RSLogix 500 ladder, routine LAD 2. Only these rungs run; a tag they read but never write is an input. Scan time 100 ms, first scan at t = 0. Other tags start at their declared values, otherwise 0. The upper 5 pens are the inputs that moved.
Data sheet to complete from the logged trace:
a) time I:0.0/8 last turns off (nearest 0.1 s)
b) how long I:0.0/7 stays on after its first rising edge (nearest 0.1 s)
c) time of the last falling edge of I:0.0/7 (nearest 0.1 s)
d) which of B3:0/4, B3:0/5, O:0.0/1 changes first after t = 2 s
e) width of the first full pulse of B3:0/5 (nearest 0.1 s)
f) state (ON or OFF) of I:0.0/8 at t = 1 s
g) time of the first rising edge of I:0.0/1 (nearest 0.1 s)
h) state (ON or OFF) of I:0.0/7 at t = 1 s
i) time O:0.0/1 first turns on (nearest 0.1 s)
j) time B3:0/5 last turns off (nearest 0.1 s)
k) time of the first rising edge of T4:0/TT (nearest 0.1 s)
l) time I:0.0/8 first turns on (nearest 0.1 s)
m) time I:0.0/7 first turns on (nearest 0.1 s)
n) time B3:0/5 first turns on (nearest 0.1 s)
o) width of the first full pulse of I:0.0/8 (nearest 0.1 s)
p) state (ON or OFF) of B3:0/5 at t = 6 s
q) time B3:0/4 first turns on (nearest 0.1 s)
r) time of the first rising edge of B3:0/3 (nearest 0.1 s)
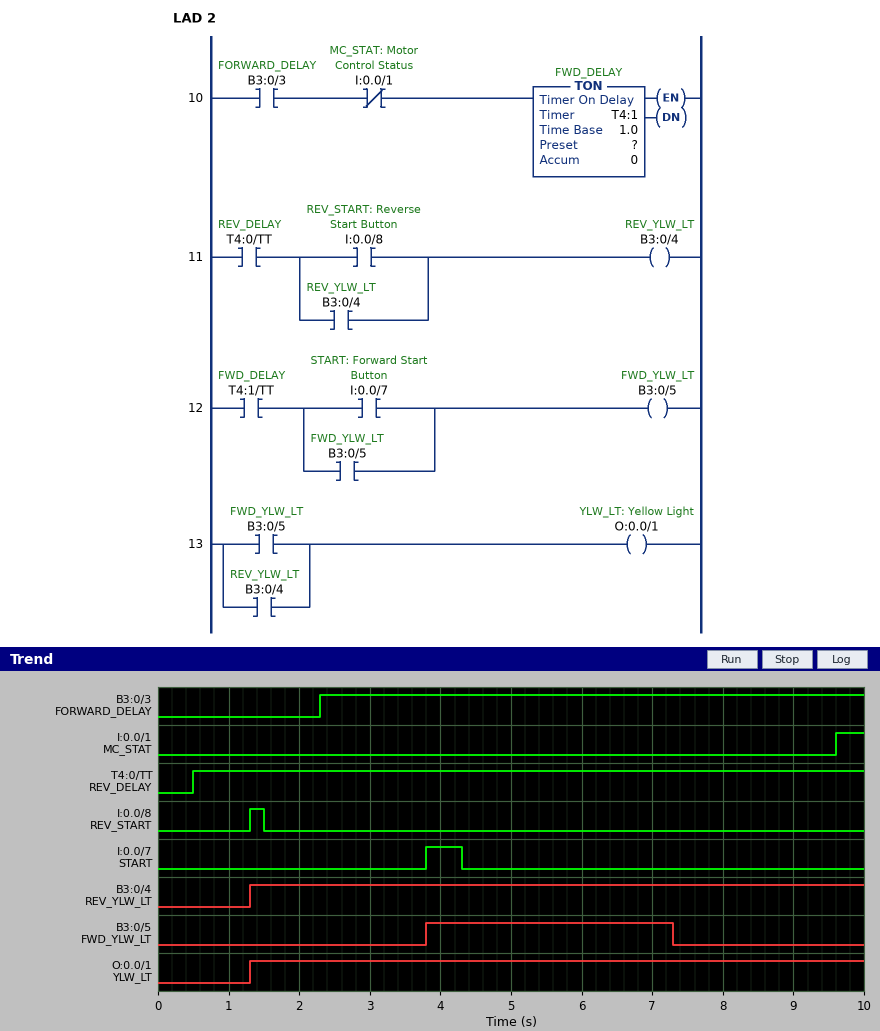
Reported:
1.5 s
0.5 s
4.3 s
B3:0/5
3.5 s
OFF
9.6 s
OFF
1.3 s
7.3 s
0.5 s
1.3 s
3.8 s
3.8 s
0.2 s
ON
1.3 s
2.3 s
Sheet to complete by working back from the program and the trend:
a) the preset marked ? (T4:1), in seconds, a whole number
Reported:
5 s
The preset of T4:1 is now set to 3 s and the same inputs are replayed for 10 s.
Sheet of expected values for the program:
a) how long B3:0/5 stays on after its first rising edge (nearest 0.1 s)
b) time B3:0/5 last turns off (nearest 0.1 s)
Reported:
1.5 s
5.3 s
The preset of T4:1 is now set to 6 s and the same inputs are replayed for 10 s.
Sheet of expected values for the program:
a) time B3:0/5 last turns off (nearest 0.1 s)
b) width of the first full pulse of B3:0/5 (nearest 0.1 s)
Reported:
8.3 s
4.5 s
